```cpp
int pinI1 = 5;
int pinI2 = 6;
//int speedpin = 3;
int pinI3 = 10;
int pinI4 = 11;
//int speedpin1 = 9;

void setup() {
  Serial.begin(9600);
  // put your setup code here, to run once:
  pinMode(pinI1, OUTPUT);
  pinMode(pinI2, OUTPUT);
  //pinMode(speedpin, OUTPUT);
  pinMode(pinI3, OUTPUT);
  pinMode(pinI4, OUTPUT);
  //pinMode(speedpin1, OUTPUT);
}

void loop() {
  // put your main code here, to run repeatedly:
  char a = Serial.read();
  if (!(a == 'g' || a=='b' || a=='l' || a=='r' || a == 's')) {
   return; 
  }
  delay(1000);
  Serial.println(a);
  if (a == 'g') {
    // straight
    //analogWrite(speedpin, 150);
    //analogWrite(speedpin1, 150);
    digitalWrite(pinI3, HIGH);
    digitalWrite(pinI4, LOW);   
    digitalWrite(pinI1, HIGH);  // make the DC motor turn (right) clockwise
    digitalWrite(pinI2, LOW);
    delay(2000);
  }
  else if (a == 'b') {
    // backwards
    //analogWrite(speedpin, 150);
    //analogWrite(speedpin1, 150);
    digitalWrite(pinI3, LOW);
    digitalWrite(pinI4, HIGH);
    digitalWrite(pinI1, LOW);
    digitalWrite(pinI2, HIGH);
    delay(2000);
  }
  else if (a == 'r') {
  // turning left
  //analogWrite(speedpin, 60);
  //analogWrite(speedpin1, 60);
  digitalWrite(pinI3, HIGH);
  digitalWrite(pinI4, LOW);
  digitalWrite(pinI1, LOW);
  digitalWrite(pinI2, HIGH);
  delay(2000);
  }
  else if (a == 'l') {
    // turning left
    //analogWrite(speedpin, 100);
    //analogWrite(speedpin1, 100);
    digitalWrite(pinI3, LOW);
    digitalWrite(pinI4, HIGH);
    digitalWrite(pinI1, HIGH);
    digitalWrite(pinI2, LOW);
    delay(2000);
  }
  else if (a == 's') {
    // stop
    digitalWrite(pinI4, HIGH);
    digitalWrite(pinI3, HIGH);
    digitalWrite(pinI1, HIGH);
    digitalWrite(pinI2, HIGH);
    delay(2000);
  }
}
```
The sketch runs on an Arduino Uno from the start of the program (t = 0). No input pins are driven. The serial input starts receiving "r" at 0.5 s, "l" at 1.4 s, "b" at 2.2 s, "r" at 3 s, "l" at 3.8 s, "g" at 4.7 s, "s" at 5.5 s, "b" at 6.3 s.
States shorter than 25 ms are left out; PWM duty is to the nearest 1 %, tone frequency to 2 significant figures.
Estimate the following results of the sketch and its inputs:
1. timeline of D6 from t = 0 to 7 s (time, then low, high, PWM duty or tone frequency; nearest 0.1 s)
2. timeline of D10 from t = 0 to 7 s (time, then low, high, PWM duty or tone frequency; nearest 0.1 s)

0 s low; 1.5 s high; 4.5 s low
0 s low; 1.5 s high; 4.5 s low
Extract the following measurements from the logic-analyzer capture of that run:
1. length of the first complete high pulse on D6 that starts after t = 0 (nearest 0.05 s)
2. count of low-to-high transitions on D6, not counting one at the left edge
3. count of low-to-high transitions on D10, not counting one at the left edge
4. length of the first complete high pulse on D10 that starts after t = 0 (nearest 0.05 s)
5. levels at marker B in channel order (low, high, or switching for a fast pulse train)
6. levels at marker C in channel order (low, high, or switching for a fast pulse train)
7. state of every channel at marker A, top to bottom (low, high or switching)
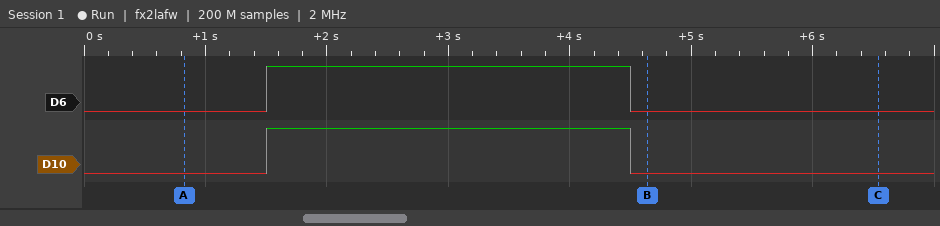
3.00 s
1
1
3.00 s
D6 low, D10 low
D6 low, D10 low
D6 low, D10 low
